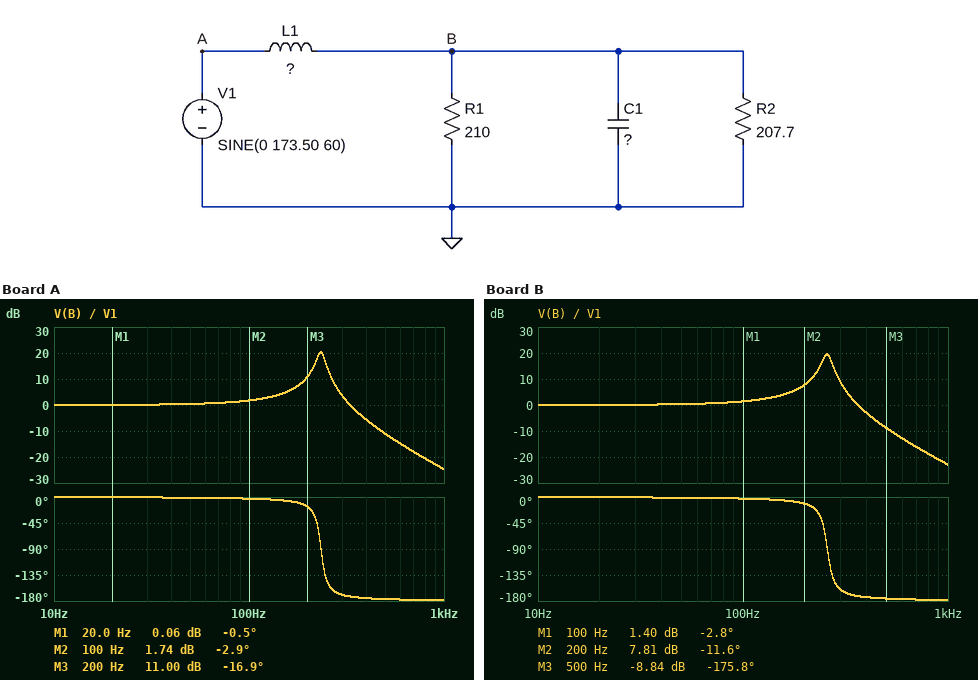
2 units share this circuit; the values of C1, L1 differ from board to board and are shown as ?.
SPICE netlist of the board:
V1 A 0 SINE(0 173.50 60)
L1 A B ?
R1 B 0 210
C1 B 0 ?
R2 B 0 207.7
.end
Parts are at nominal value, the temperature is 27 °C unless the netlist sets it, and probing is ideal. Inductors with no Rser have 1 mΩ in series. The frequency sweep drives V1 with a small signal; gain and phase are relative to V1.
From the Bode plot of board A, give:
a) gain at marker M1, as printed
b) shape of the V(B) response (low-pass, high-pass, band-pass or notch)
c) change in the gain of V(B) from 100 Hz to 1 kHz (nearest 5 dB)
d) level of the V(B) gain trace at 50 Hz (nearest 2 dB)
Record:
0.06 dB
low-pass
-25 dB
0 dB
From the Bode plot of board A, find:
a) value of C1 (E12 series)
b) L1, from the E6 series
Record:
68 µF
6.8 mH
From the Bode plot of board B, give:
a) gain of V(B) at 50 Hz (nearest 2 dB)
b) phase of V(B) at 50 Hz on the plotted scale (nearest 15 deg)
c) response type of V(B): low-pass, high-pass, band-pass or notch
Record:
0 dB
0 deg
low-pass
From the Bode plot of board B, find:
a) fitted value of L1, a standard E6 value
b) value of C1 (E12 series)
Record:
6.8 mH
56 µF
